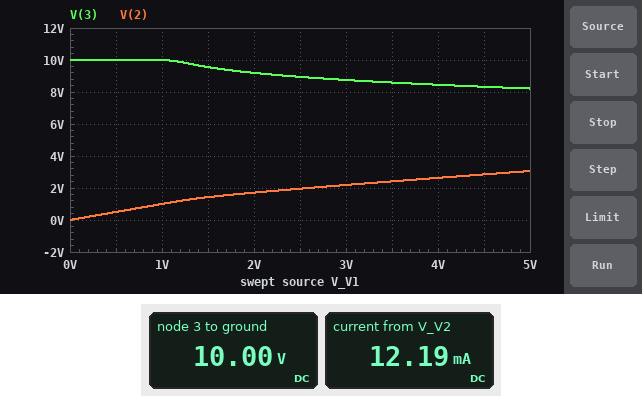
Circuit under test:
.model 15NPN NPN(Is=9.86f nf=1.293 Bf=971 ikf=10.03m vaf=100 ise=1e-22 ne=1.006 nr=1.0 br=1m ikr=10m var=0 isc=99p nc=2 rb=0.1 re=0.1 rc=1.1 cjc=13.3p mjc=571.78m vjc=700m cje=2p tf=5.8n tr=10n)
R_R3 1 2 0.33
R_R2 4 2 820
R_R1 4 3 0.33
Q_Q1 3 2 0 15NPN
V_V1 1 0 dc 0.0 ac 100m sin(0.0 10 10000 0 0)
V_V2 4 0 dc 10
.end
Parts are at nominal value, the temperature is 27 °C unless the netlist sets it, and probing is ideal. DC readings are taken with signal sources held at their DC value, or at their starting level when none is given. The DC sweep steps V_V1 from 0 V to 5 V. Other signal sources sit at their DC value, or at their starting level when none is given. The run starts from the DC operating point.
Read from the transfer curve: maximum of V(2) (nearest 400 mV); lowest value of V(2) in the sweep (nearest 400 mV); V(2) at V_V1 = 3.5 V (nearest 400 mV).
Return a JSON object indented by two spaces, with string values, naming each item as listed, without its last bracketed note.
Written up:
{
  "maximum of V(2)": "3.2 V",
  "lowest value of V(2) in the sweep": "0 V",
  "V(2) at V_V1 = 3.5 V": "2.4 V"
}
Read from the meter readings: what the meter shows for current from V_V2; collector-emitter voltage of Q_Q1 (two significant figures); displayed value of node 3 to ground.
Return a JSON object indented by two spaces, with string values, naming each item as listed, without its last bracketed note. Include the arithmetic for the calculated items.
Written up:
{
  "what the meter shows for current from V_V2": "12.19 mA",
  "collector-emitter voltage of Q_Q1": "10 V = 10 V",
  "displayed value of node 3 to ground": "10.00 V"
}
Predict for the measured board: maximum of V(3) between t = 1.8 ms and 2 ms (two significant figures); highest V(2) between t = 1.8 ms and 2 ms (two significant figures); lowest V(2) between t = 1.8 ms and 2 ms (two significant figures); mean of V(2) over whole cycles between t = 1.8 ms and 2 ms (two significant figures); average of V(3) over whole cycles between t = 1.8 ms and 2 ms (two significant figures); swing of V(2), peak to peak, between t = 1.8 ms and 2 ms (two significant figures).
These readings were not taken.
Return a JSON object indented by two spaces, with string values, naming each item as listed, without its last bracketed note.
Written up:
{
  "maximum of V(3) between t = 1.8 ms and 2 ms": "10 V",
  "highest V(2) between t = 1.8 ms and 2 ms": "4.9 V",
  "lowest V(2) between t = 1.8 ms and 2 ms": "-10 V",
  "mean of V(2) over whole cycles between t = 1.8 ms and 2 ms": "-1.4 V",
  "average of V(3) over whole cycles between t = 1.8 ms and 2 ms": "9.3 V",
  "swing of V(2), peak to peak, between t = 1.8 ms and 2 ms": "15 V"
}
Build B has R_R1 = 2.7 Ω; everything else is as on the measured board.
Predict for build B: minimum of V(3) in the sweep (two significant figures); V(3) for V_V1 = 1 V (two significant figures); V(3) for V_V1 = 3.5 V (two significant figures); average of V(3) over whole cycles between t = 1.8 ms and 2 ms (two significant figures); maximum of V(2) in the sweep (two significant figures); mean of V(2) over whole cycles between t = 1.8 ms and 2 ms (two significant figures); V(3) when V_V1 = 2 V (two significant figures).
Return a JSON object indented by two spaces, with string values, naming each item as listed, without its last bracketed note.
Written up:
{
  "minimum of V(3) in the sweep": "3.6 V",
  "V(3) for V_V1 = 1 V": "9.9 V",
  "V(3) for V_V1 = 3.5 V": "3.8 V",
  "average of V(3) over whole cycles between t = 1.8 ms and 2 ms": "7.4 V",
  "maximum of V(2) in the sweep": "2.9 V",
  "mean of V(2) over whole cycles between t = 1.8 ms and 2 ms": "-1.5 V",
  "V(3) when V_V1 = 2 V": "3.7 V"
}
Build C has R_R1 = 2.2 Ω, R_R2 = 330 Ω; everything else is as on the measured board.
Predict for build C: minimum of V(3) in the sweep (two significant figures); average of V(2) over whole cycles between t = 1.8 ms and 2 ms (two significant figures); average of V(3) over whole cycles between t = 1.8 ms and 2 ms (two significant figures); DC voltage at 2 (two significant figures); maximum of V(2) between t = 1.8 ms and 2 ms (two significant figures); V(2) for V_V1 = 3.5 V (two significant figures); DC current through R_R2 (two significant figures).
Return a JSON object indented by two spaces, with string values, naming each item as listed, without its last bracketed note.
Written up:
{
  "minimum of V(3) in the sweep": "4.1 V",
  "average of V(2) over whole cycles between t = 1.8 ms and 2 ms": "-1.5 V",
  "average of V(3) over whole cycles between t = 1.8 ms and 2 ms": "7.6 V",
  "DC voltage at 2": "10 mV",
  "maximum of V(2) between t = 1.8 ms and 2 ms": "4.8 V",
  "V(2) for V_V1 = 3.5 V": "2.3 V",
  "DC current through R_R2": "30 mA"
}
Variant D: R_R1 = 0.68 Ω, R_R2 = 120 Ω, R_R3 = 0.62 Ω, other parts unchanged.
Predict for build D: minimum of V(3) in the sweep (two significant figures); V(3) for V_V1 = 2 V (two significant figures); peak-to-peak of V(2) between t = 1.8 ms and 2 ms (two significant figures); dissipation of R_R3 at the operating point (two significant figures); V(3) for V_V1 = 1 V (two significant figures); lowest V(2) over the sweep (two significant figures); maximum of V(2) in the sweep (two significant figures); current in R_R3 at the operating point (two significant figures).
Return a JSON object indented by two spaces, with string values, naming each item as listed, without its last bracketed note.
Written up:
{
  "minimum of V(3) in the sweep": "6.9 V",
  "V(3) for V_V1 = 2 V": "8.5 V",
  "peak-to-peak of V(2) between t = 1.8 ms and 2 ms": "14 V",
  "dissipation of R_R3 at the operating point": "4.3 mW",
  "V(3) for V_V1 = 1 V": "10 V",
  "lowest V(2) over the sweep": "51 mV",
  "maximum of V(2) in the sweep": "2.6 V",
  "current in R_R3 at the operating point": "83 mA"
}
